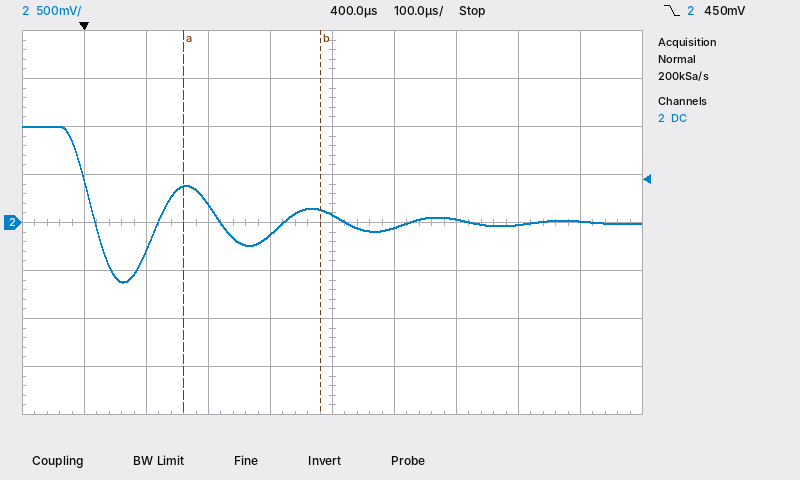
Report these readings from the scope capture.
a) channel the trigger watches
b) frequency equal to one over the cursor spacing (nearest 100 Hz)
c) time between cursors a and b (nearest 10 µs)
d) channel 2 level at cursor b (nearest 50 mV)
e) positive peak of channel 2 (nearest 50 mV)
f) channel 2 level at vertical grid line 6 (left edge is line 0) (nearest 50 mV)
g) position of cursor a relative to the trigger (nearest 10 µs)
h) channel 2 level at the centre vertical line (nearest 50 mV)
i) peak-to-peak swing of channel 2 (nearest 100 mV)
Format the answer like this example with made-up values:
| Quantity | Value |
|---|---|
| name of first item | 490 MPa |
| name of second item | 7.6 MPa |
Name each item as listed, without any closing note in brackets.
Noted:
| Quantity | Value |
|---|---|
| channel the trigger watches | channel 2 |
| frequency equal to one over the cursor spacing | 4.5 kHz |
| time between cursors a and b | 220 µs |
| channel 2 level at cursor b | 150 mV |
| positive peak of channel 2 | 1.00 V |
| channel 2 level at vertical grid line 6 (left edge is line 0) | -50 mV |
| position of cursor a relative to the trigger | +160 µs |
| channel 2 level at the centre vertical line | 100 mV |
| peak-to-peak swing of channel 2 | 1.60 V |
